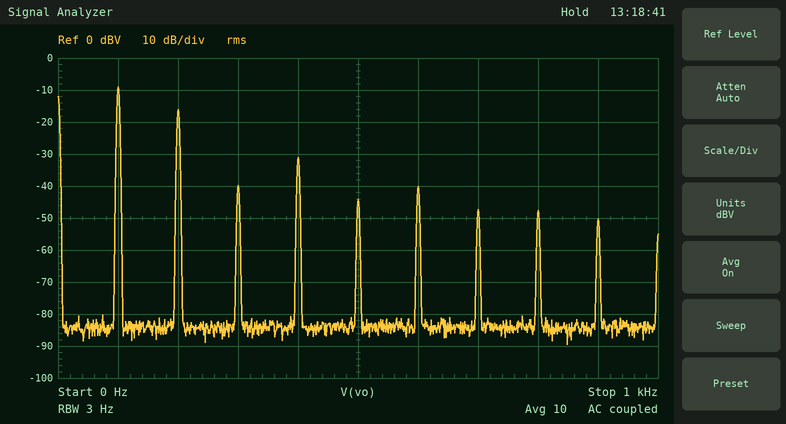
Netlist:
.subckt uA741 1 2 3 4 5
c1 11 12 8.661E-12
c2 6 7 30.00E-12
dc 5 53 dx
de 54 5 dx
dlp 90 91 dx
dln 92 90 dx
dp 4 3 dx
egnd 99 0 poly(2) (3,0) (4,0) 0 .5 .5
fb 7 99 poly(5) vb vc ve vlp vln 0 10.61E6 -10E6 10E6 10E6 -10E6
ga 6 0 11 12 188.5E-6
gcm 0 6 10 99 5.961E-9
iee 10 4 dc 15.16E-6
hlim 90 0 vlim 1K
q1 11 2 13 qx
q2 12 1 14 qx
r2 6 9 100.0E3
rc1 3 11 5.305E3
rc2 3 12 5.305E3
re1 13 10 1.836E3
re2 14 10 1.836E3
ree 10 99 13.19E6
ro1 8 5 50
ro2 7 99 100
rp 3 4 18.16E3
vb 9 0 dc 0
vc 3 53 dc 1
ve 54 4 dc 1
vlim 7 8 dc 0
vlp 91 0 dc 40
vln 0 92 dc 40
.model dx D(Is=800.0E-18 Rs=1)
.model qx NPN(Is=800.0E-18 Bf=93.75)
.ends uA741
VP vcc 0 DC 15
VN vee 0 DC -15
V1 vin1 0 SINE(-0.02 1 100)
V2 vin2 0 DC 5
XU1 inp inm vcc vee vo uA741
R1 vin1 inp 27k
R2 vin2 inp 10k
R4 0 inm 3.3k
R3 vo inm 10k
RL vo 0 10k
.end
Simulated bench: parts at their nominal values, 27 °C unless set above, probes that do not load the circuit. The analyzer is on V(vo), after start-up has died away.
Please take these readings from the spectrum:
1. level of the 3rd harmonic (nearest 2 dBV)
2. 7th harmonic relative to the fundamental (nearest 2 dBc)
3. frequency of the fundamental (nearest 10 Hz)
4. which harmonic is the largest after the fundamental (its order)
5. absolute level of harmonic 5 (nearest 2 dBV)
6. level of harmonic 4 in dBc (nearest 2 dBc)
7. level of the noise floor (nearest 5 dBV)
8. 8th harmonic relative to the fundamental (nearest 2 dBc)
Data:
-40 dBV
-38 dBc
100 Hz
2
-44 dBV
-22 dBc
-85 dBV
-38 dBc
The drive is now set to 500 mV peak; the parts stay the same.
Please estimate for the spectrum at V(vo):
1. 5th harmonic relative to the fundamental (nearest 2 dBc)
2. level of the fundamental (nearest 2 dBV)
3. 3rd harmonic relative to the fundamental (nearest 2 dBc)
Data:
-30 dBc
-16 dBV
-24 dBc
